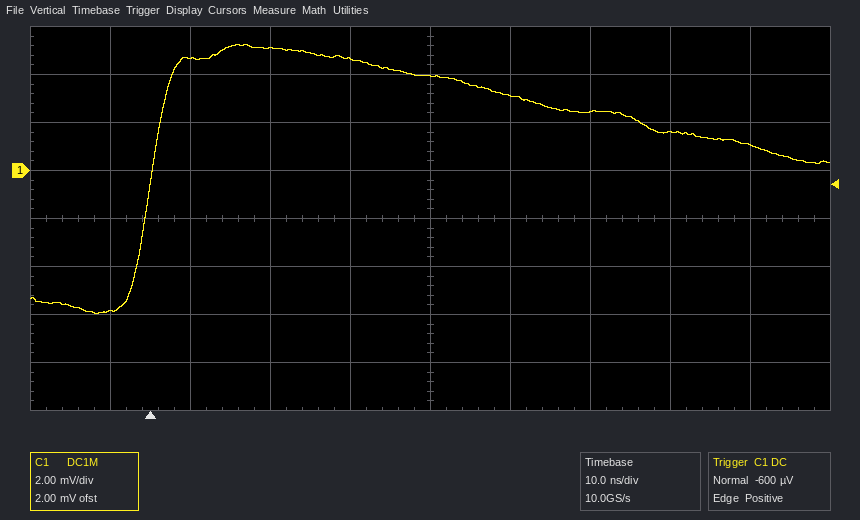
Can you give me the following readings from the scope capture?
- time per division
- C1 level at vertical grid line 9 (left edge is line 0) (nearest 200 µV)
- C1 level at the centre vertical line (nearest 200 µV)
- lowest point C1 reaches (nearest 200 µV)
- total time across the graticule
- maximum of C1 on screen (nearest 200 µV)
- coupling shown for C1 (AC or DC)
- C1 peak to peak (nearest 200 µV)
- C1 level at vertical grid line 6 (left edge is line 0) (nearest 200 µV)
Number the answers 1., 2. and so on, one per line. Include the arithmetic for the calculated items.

1. 10 ns
2. 1.0 mV
3. 4.0 mV
4. -6.0 mV
5. 100 ns
6. 5.2 mV
7. DC
8. 5.2 mV − (-6.0 mV) = 11.2 mV
9. 3.2 mV
